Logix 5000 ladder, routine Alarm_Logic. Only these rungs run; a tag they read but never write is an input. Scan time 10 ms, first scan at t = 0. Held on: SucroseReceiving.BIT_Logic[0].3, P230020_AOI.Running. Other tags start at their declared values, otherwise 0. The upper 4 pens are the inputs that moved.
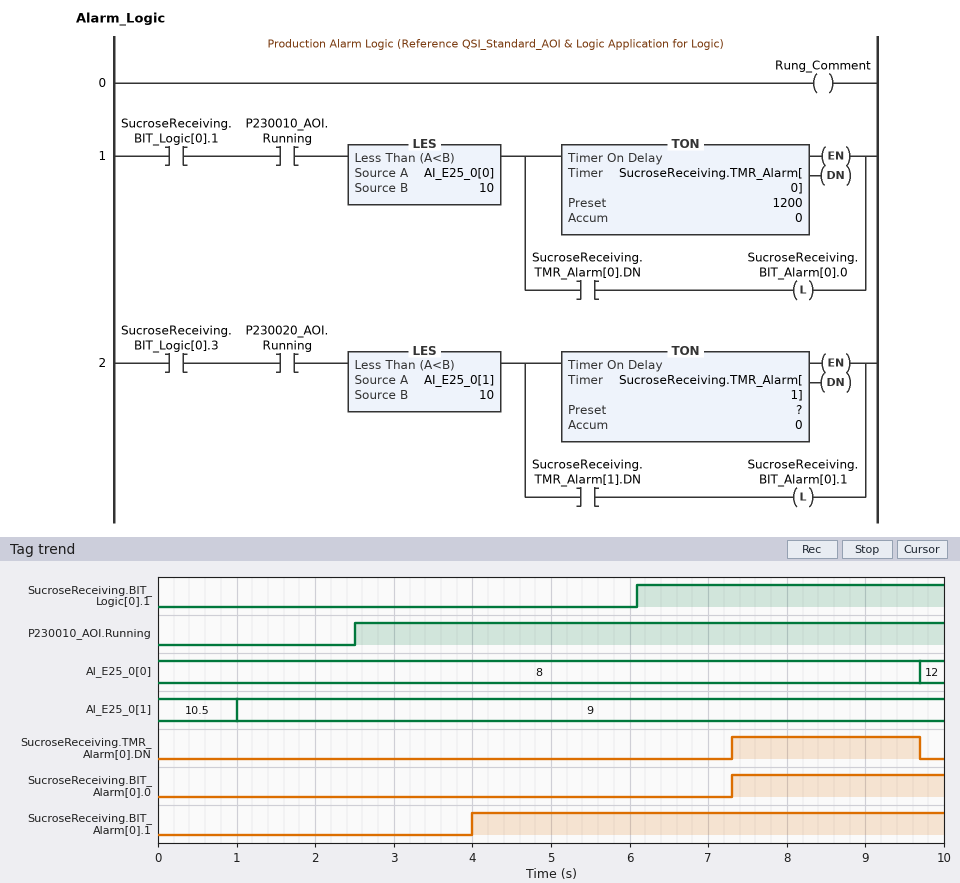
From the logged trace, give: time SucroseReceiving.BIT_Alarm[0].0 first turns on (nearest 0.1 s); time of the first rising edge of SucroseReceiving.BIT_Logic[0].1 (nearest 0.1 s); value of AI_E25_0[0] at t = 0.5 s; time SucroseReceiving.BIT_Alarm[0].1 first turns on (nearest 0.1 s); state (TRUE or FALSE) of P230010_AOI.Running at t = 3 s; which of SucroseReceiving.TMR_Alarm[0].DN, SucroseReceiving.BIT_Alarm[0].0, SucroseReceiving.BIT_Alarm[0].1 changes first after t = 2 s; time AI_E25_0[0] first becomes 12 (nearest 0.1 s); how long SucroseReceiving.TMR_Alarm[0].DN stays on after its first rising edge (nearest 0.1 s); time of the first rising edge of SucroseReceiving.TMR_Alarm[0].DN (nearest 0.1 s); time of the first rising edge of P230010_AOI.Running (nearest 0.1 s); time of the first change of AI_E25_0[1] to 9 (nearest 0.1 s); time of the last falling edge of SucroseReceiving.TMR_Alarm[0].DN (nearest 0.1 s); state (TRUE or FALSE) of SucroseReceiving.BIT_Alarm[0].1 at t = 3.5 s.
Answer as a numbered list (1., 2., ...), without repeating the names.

1. 7.3 s
2. 6.1 s
3. 8
4. 4.0 s
5. TRUE
6. SucroseReceiving.BIT_Alarm[0].1
7. 9.7 s
8. 2.4 s
9. 7.3 s
10. 2.5 s
11. 1.0 s
12. 9.7 s
13. FALSE
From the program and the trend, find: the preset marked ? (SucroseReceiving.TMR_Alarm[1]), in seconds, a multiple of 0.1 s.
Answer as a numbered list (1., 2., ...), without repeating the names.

1. 3.0 s
